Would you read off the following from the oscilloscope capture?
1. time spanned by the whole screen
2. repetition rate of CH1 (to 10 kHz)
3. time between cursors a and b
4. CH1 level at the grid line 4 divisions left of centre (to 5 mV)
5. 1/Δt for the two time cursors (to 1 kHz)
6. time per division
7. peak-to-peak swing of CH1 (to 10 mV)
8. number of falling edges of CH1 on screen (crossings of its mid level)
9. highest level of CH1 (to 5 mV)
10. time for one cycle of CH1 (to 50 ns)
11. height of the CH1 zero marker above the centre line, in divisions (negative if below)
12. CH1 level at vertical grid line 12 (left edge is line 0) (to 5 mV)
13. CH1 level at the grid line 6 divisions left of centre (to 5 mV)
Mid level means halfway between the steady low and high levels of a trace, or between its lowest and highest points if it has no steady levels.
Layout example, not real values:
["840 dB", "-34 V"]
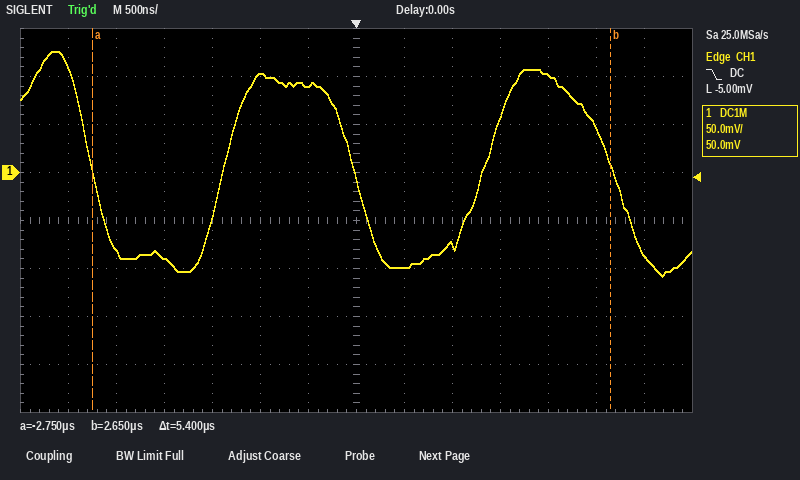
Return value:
["7 µs", "370 kHz", "5.4 µs", "-90 mV", "185 kHz", "500 ns", "230 mV", "3", "125 mV", "2.70 µs", "+1.0 div", "45 mV", "110 mV"]
